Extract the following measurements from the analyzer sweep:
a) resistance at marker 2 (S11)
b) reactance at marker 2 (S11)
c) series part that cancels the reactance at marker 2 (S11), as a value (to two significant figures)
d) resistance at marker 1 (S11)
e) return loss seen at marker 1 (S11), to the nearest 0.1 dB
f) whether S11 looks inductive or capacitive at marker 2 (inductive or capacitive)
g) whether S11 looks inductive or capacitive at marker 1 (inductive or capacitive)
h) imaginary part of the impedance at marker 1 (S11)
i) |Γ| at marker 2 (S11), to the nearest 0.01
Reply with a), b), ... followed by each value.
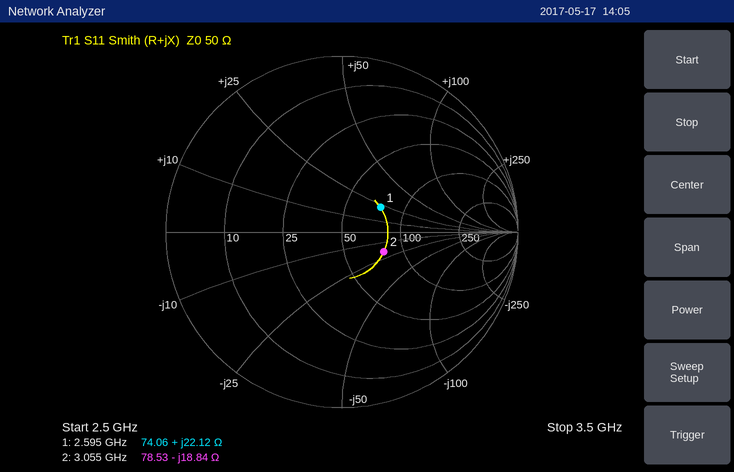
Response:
a) 78.53 Ω
b) -18.84 Ω
c) 980 pH
d) 74.06 Ω
e) 11.7 dB
f) capacitive
g) inductive
h) +22.12 Ω
i) 0.26
